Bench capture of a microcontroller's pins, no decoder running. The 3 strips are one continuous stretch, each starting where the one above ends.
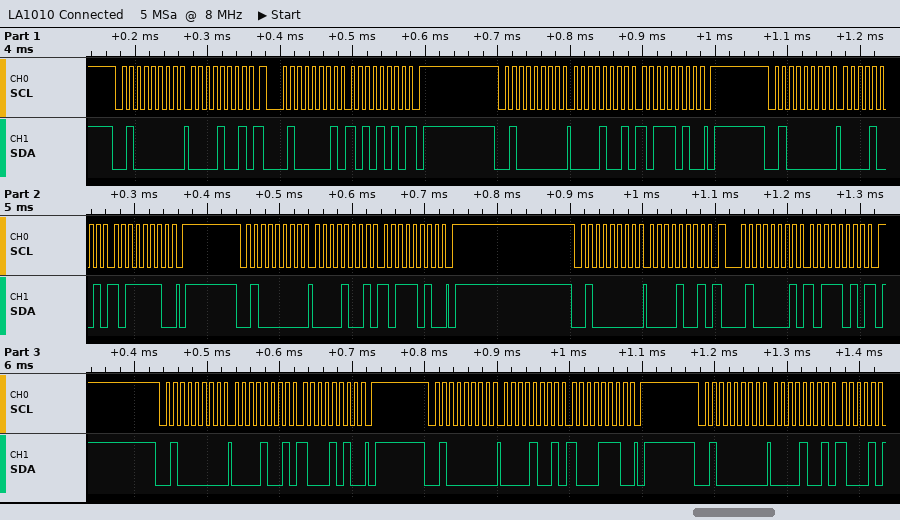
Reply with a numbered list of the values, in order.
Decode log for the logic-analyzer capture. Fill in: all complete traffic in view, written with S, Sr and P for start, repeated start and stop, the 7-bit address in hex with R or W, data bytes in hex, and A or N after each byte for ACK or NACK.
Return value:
1. S 20W A 09 A Sr 20R A AA N P S 20W A 09 A BA A P S 20W A 09 A BE A P S 20W A 09 A BA A P S 20W A 09 A Sr 20R A BA N P S 20W A 09 A 8A A P S 20W A 09 A 8E A P S 20W A 09 A
